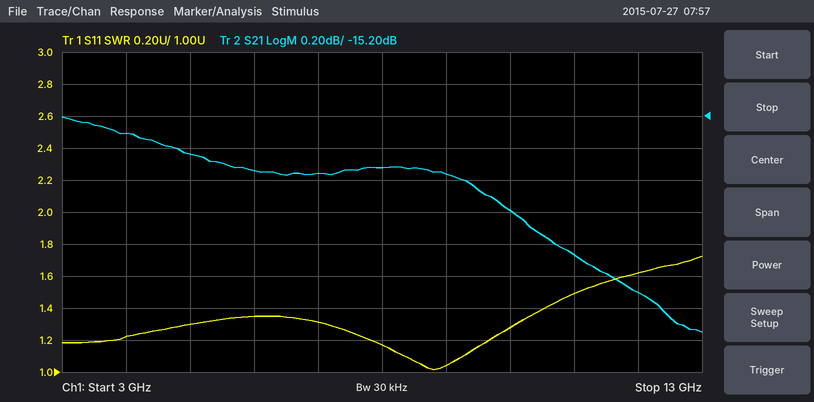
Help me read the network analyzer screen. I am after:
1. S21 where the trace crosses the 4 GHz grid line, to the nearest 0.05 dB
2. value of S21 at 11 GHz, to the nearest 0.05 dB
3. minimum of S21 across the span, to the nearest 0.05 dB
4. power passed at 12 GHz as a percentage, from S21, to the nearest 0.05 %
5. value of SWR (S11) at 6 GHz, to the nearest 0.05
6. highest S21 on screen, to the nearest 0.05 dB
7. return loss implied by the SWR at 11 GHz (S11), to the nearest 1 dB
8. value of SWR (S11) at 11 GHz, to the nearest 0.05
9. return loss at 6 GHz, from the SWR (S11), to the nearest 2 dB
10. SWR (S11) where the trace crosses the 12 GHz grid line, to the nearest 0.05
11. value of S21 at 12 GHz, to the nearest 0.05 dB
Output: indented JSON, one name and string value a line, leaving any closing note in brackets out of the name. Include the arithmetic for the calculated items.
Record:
{
  "S21 where the trace crosses the 4 GHz grid line, to the nearest 0.05 dB": "-15.30 dB",
  "value of S21 at 11 GHz, to the nearest 0.05 dB": "-16.05 dB",
  "minimum of S21 across the span, to the nearest 0.05 dB": "-16.55 dB",
  "power passed at 12 GHz as a percentage, from S21, to the nearest 0.05 %": "10^(-16.3/10) ≈ 2.34 %, so 2.35 % to the nearest 0.05 %",
  "value of SWR (S11) at 6 GHz, to the nearest 0.05": "1.35",
  "highest S21 on screen, to the nearest 0.05 dB": "-15.20 dB",
  "return loss implied by the SWR at 11 GHz (S11), to the nearest 1 dB": "−20 log10((1.5 − 1)/(1.5 + 1)) ≈ 14 dB",
  "value of SWR (S11) at 11 GHz, to the nearest 0.05": "1.50",
  "return loss at 6 GHz, from the SWR (S11), to the nearest 2 dB": "−20 log10((1.35 − 1)/(1.35 + 1)) ≈ 16 dB",
  "SWR (S11) where the trace crosses the 12 GHz grid line, to the nearest 0.05": "1.60",
  "value of S21 at 12 GHz, to the nearest 0.05 dB": "-16.30 dB"
}
